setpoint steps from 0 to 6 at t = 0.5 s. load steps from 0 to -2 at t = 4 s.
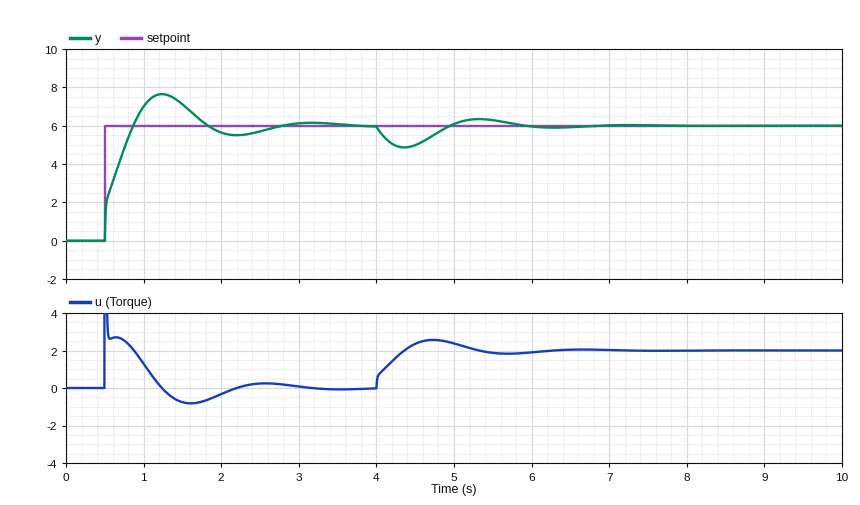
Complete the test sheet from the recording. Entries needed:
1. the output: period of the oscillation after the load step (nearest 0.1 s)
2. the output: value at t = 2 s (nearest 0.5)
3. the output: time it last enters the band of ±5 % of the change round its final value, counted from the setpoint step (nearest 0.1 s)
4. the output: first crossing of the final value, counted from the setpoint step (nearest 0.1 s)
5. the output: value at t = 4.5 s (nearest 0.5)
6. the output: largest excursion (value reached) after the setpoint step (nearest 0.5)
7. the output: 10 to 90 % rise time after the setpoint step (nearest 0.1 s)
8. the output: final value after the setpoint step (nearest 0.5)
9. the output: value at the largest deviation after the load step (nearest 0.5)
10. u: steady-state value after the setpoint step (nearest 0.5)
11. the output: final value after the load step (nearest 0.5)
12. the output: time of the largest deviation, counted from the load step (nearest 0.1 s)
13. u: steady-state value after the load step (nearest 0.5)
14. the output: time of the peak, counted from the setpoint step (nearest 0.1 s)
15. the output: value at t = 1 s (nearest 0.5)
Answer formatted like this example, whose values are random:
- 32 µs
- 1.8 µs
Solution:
- 1.9 s
- 5.5
- 2.0 s
- 0.4 s
- 5.0
- 7.5
- 0.3 s
- 6.0
- 5.0
- 0.0
- 6.0
- 0.4 s
- 2.0
- 0.7 s
- 7.0
